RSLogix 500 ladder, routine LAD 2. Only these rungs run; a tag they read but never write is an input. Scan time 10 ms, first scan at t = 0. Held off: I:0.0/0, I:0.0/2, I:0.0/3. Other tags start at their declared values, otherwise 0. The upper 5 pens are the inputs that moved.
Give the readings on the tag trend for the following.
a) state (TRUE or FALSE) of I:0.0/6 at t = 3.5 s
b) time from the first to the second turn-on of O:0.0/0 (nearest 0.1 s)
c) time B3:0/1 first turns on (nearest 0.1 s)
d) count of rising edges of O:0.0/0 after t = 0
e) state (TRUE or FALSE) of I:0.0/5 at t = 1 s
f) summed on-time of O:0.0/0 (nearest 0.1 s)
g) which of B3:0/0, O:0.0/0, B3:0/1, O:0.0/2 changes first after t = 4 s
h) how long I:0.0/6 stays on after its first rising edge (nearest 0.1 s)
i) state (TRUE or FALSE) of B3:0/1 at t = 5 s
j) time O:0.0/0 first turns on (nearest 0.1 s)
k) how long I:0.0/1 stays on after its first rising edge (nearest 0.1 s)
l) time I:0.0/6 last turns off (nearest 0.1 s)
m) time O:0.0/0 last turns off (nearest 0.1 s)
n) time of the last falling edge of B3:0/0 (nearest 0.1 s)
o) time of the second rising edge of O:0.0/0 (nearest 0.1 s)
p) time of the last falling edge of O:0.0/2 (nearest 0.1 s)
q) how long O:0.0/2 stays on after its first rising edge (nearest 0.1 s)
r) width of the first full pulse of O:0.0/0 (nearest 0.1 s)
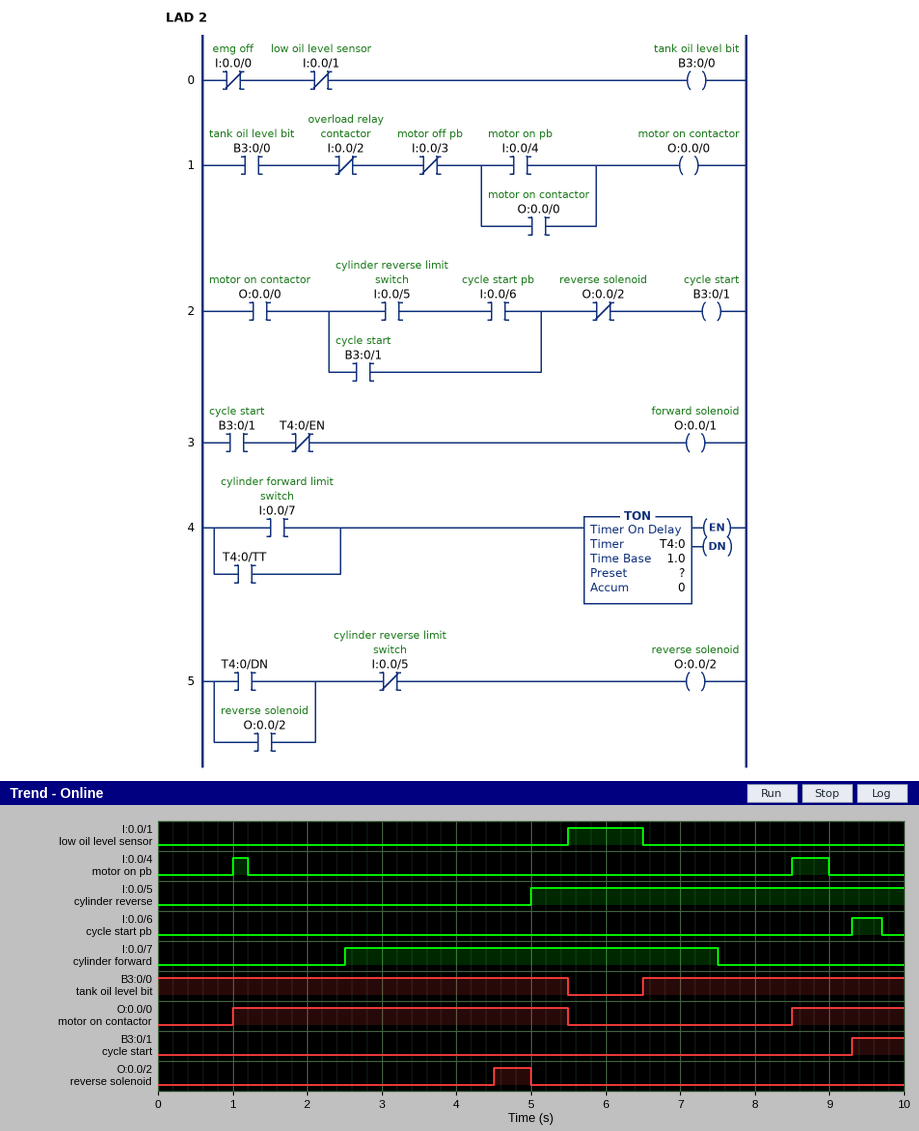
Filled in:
FALSE
7.5 s
9.3 s
2
FALSE
6.0 s
O:0.0/2
0.4 s
FALSE
1.0 s
1.0 s
9.7 s
5.5 s
5.5 s
8.5 s
5.0 s
0.5 s
4.5 s
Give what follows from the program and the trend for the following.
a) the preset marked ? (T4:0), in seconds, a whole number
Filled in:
2 s
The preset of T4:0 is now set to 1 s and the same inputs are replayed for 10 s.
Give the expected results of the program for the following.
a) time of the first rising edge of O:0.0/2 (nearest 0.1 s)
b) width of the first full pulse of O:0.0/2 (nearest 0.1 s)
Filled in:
3.5 s
1.5 s
